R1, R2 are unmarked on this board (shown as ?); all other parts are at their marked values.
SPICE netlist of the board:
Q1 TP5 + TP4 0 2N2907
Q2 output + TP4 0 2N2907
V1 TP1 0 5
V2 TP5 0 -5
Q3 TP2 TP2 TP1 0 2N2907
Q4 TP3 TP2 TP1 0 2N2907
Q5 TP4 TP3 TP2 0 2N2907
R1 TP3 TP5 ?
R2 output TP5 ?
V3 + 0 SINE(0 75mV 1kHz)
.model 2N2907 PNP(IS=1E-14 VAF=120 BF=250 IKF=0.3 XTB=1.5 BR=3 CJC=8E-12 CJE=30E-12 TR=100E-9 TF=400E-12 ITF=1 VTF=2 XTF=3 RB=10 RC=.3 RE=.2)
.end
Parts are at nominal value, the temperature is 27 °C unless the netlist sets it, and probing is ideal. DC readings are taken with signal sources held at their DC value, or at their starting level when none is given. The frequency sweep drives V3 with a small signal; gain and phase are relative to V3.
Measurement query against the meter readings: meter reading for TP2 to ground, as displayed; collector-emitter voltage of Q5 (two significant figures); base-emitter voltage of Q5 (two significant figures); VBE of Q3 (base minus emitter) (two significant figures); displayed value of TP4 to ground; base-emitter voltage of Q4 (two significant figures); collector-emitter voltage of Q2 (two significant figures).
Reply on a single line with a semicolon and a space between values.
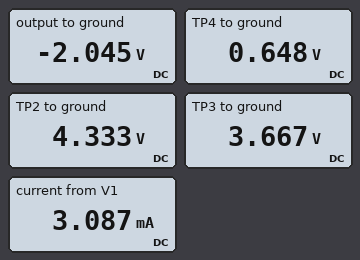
4.333 V; -3.7 V; -670 mV; -670 mV; 0.648 V; -670 mV; -2.7 V
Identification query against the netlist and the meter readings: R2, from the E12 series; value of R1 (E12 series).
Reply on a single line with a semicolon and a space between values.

3.9 kΩ; 5.6 kΩ
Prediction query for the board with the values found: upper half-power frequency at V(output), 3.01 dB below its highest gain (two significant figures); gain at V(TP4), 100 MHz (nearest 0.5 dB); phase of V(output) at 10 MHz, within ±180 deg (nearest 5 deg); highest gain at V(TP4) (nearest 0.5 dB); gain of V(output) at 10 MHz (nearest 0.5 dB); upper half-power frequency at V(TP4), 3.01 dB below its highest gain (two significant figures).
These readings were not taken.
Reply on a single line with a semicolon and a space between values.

4.2 GHz; -0.5 dB; 75 deg; 0 dB; -17.0 dB; 3.4 GHz
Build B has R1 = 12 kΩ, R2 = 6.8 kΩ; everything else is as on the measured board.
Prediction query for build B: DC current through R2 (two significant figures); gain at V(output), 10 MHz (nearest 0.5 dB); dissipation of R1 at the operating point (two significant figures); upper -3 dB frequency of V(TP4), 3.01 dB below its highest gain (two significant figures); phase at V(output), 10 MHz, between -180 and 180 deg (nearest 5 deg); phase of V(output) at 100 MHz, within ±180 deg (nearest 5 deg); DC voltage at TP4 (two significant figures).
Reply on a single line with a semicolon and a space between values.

360 µA; -12.0 dB; 6.3 mW; 3.5 GHz; 90 deg; 15 deg; 630 mV
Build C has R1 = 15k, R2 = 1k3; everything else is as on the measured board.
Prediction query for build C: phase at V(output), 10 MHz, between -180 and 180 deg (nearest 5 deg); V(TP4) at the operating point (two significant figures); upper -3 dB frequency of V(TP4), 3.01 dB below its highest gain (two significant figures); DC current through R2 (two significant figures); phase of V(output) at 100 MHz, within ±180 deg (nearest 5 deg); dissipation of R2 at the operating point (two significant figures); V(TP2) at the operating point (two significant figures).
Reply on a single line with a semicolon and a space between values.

160 deg; 620 mV; 3.5 GHz; 290 µA; 25 deg; 110 µW; 4.4 V
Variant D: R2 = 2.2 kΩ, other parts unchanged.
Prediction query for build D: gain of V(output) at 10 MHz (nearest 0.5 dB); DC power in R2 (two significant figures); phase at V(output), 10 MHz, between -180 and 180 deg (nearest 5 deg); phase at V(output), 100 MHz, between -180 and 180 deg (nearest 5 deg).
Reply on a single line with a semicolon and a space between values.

-22.5 dB; 1.3 mW; 135 deg; 40 deg
